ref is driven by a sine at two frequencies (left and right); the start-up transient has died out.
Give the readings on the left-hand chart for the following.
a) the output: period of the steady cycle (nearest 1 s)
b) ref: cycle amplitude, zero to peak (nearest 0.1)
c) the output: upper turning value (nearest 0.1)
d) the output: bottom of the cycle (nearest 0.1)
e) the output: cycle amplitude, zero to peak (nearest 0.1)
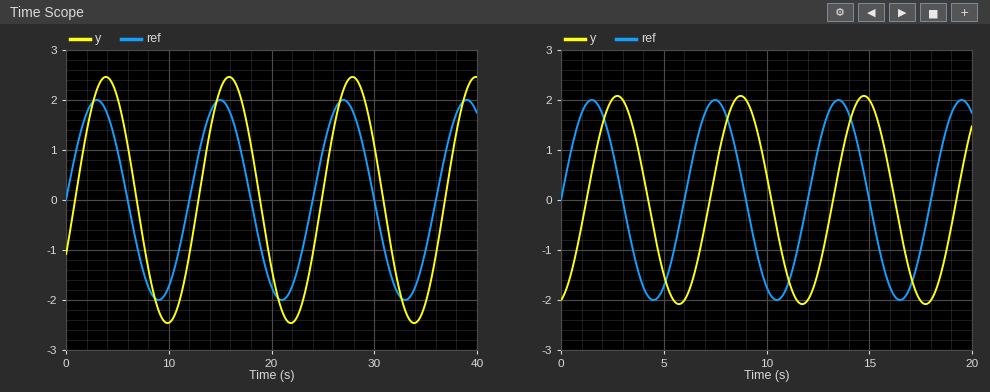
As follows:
12 s
2.0
2.5
-2.5
2.5
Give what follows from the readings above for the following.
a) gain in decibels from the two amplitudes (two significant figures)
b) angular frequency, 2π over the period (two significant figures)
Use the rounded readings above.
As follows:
1.9 dB
0.52 rad/s
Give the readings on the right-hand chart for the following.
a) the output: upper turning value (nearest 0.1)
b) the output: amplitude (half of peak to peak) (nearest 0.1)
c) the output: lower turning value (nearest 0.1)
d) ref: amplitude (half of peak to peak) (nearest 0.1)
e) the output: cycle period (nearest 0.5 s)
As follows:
2.1
2.1
-2.1
2.0
6.0 s
